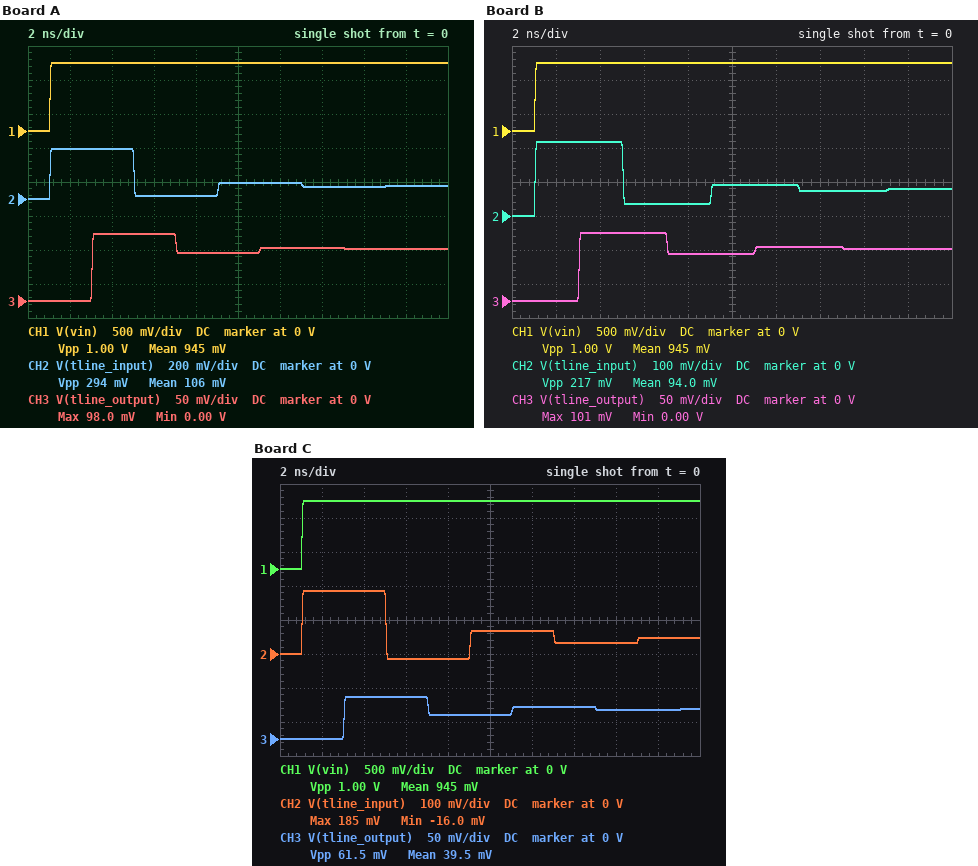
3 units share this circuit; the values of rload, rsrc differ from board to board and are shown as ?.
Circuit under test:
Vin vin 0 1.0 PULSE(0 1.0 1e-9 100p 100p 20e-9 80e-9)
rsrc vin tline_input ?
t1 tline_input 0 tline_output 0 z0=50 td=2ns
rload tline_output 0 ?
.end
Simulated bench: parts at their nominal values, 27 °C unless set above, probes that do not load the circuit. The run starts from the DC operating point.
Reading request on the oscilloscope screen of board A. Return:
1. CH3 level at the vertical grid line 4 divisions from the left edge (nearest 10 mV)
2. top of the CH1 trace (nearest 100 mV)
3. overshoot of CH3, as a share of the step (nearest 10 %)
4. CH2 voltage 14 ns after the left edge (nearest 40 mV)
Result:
70 mV
1.0 V
30 %
80 mV
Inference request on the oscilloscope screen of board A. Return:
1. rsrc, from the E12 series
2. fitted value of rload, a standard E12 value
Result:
120 Ω
10 Ω
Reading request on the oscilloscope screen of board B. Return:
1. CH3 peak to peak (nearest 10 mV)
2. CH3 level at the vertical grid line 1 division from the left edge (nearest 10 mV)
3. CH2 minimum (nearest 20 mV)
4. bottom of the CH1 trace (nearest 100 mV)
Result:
100 mV
0 V
0 V
0 V
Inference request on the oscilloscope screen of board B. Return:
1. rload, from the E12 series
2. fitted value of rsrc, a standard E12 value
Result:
15 Ω
180 Ω
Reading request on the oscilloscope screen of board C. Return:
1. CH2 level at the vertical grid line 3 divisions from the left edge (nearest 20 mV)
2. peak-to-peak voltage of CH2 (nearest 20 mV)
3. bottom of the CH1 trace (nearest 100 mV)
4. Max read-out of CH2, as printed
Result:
-20 mV
200 mV
0 V
185 mV
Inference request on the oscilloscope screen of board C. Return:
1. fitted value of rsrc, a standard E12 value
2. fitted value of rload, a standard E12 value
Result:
220 Ω
10 Ω
